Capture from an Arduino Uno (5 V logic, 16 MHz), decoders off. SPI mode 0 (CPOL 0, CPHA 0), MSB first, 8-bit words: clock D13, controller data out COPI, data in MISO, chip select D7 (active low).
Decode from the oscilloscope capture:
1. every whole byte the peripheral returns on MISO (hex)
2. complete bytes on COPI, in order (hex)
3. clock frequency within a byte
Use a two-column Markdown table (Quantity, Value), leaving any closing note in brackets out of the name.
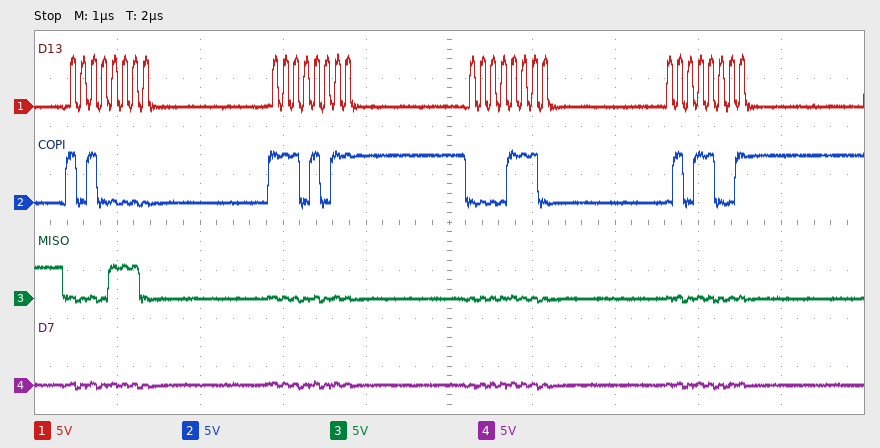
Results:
| Quantity | Value |
|---|---|
| every whole byte the peripheral returns on MISO | 0E 00 00 00 |
| complete bytes on COPI, in order | A0 EB 0E 59 |
| clock frequency within a byte | 8 MHz |
